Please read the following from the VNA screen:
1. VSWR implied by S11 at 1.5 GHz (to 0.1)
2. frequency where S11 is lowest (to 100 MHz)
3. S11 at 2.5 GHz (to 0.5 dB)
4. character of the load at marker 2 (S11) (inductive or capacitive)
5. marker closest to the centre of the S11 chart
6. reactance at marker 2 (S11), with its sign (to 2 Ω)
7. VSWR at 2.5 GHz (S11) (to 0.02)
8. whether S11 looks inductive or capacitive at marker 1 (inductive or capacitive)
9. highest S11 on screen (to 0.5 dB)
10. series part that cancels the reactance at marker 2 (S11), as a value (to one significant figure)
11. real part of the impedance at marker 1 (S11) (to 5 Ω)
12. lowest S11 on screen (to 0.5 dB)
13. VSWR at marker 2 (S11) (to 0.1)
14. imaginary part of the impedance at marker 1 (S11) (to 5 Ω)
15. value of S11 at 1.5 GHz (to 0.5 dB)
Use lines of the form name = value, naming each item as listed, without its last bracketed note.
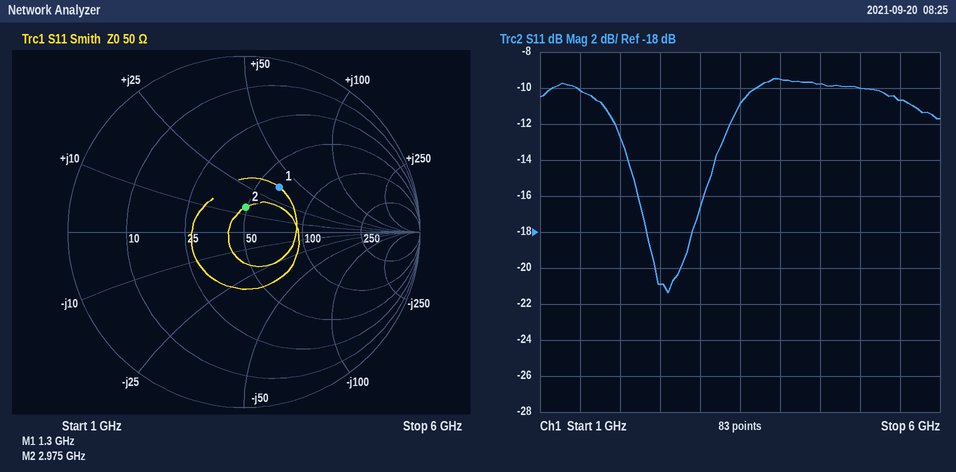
VSWR implied by S11 at 1.5 GHz = 1.9
frequency where S11 is lowest = 2.6 GHz
S11 at 2.5 GHz = -21.0 dB
character of the load at marker 2 (S11) = inductive
marker closest to the centre of the S11 chart = marker 2
reactance at marker 2 (S11), with its sign = +14 Ω
VSWR at 2.5 GHz (S11) = 1.20
whether S11 looks inductive or capacitive at marker 1 = inductive
highest S11 on screen = -9.5 dB
series part that cancels the reactance at marker 2 (S11), as a value = 4 pF
real part of the impedance at marker 1 (S11) = 65 Ω
lowest S11 on screen = -21.5 dB
VSWR at marker 2 (S11) = 1.3
imaginary part of the impedance at marker 1 (S11) = +35 Ω
value of S11 at 1.5 GHz = -10.0 dB
